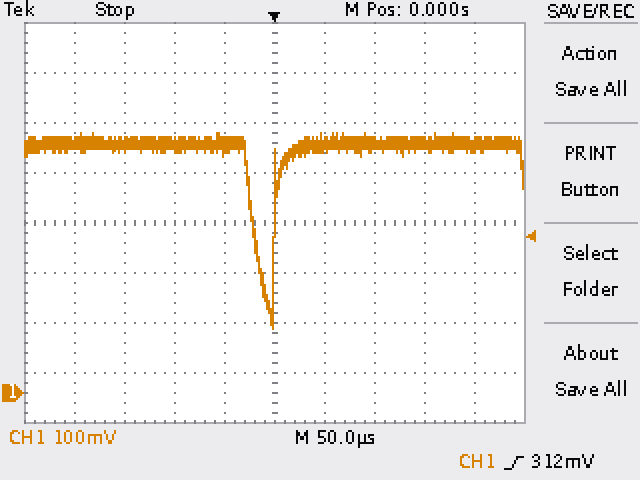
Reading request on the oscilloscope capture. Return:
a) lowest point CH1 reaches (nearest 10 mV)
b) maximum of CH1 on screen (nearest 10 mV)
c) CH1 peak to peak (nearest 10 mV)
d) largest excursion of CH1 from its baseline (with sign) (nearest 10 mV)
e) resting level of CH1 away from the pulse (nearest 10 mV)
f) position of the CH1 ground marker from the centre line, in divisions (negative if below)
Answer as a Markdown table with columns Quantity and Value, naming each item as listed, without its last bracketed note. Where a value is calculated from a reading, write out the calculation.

| Quantity | Value |
|---|---|
| lowest point CH1 reaches | 130 mV |
| maximum of CH1 on screen | 520 mV |
| CH1 peak to peak | 520 mV − (130 mV) = 390 mV |
| largest excursion of CH1 from its baseline (with sign) | 130 mV − (500 mV) = -370 mV |
| resting level of CH1 away from the pulse | 500 mV |
| position of the CH1 ground marker from the centre line, in divisions | -3.4 div |
